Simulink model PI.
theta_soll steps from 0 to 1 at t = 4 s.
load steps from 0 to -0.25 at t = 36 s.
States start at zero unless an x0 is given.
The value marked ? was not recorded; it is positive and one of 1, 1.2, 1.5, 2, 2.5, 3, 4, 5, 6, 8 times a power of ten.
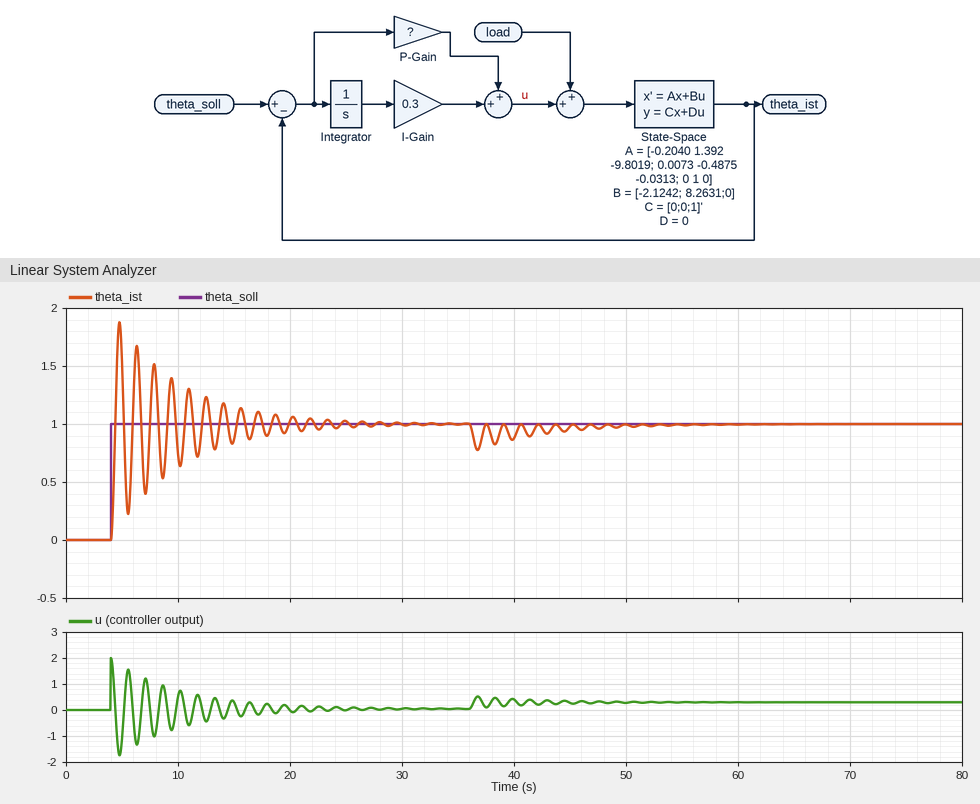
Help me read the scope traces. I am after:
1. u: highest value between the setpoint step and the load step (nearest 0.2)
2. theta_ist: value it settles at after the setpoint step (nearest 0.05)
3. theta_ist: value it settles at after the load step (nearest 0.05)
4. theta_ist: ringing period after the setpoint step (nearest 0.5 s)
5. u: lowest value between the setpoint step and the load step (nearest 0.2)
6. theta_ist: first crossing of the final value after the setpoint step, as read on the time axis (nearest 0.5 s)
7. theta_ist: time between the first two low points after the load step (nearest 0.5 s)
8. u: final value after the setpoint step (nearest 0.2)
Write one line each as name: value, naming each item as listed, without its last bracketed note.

u: highest value between the setpoint step and the load step: 2.0
theta_ist: value it settles at after the setpoint step: 1.00
theta_ist: value it settles at after the load step: 1.00
theta_ist: ringing period after the setpoint step: 1.5 s
u: lowest value between the setpoint step and the load step: -1.8
theta_ist: first crossing of the final value after the setpoint step, as read on the time axis: 4.5 s
theta_ist: time between the first two low points after the load step: 1.5 s
u: final value after the setpoint step: 0.0
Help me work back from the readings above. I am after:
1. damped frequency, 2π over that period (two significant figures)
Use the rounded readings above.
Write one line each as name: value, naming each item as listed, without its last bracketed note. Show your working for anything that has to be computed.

damped frequency, 2π over that period: 2π / 1.5 = 4.2 rad/s
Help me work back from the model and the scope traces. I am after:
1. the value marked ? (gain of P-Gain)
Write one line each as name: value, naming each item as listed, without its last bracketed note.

the value marked ?: 2
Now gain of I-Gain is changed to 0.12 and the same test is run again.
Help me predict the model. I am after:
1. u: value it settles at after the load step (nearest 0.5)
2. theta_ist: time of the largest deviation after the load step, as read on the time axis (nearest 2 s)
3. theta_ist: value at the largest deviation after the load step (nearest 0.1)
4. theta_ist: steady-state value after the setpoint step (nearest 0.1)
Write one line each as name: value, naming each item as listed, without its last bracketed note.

u: value it settles at after the load step: 0.5
theta_ist: time of the largest deviation after the load step, as read on the time axis: 36 s
theta_ist: value at the largest deviation after the load step: 0.8
theta_ist: steady-state value after the setpoint step: 1.0
